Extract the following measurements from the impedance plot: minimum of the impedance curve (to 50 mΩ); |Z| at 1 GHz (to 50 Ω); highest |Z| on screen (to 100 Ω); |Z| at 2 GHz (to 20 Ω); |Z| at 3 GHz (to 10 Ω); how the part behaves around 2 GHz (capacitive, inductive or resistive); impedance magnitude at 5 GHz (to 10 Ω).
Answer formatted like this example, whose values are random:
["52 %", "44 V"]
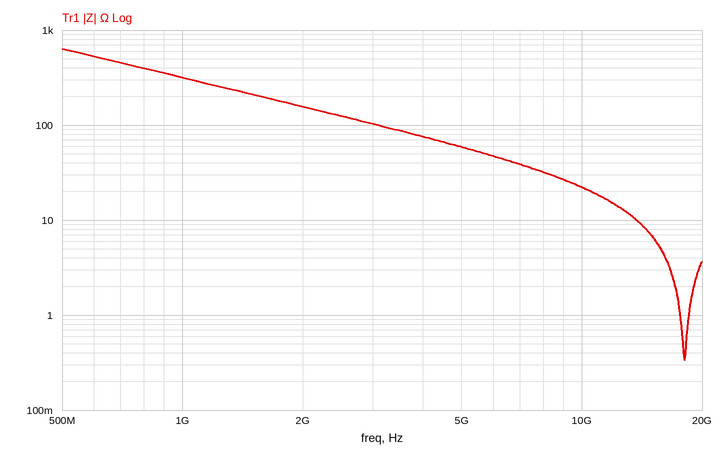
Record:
["350 mΩ", "300 Ω", "600 Ω", "160 Ω", "100 Ω", "capacitive", "60 Ω"]
